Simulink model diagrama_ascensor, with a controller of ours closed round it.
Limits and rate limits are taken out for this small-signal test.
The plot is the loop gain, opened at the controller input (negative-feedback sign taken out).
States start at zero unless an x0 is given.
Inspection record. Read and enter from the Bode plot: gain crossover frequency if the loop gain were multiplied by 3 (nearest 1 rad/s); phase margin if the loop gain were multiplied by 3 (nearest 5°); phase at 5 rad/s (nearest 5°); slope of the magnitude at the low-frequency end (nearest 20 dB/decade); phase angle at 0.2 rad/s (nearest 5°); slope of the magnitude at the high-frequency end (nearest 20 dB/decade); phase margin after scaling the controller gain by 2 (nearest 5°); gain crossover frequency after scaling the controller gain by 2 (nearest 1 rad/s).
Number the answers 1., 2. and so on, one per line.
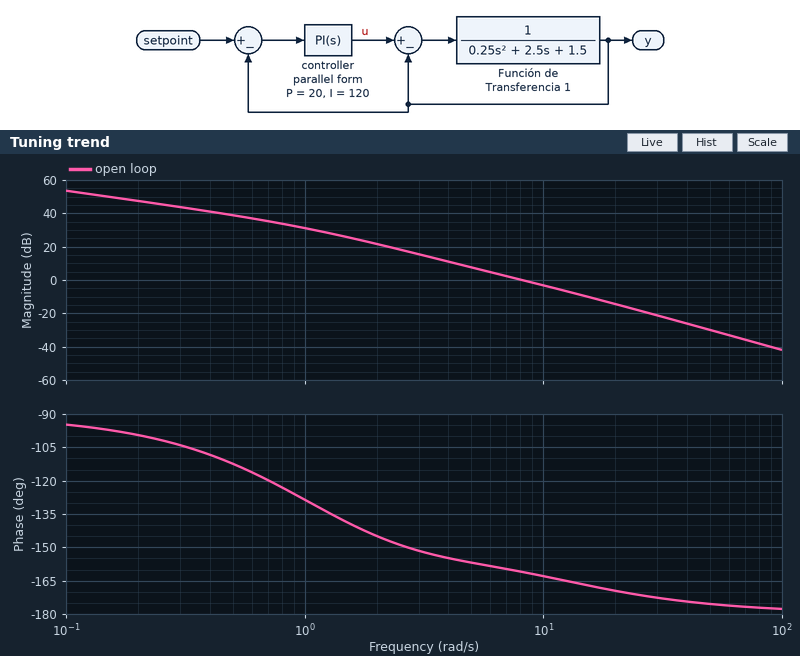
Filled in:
1. 15 rad/s
2. 15°
3. -155°
4. -20 dB/decade
5. -100°
6. -40 dB/decade
7. 15°
8. 12 rad/s
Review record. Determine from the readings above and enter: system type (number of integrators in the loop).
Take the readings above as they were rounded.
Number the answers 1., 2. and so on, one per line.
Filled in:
1. 1
